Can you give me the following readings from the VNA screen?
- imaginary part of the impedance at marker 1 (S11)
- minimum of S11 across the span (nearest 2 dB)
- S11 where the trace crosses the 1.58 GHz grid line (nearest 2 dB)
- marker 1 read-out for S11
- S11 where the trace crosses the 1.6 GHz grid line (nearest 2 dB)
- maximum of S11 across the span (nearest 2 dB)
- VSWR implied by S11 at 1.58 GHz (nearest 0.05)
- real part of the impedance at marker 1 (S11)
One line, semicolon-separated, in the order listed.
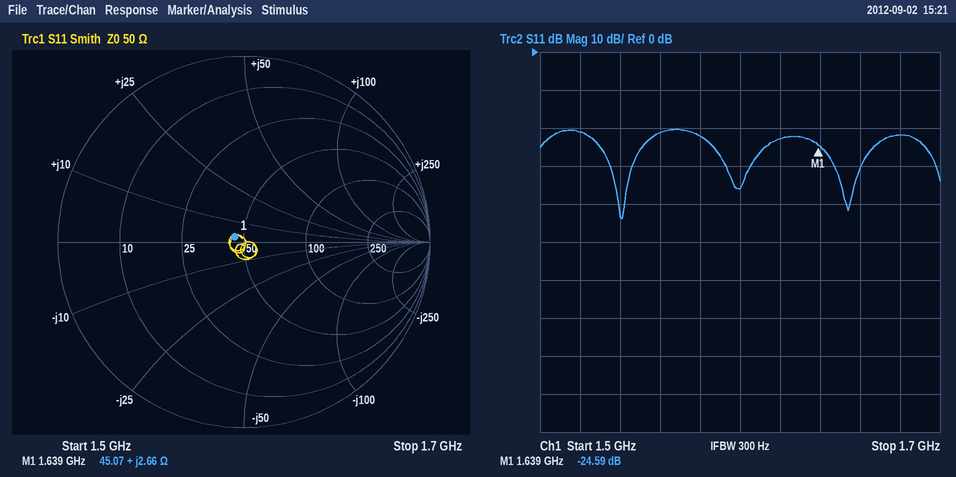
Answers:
+2.66 Ω; -44 dB; -22 dB; -24.59 dB; -36 dB; -20 dB; 1.15; 45.07 Ω
